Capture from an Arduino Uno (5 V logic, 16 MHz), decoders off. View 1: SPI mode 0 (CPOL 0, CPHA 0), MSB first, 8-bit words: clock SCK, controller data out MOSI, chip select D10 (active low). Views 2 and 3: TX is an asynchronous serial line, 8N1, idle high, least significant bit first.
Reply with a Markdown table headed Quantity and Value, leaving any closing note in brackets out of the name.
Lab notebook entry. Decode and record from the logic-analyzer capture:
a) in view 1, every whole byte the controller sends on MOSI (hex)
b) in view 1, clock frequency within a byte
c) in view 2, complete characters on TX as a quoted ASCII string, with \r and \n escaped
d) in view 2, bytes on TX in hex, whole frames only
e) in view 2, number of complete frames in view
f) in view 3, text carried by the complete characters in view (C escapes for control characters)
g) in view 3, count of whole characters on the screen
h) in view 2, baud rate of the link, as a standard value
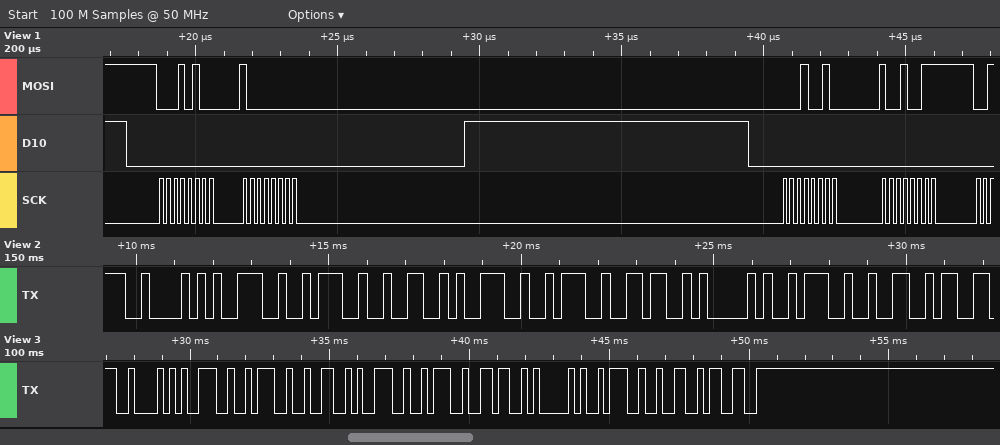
| Quantity | Value |
|---|---|
| in view 1, every whole byte the controller sends on MOSI | 14 80 12 93 |
| in view 1, clock frequency within a byte | 4 MHz |
| in view 2, complete characters on TX as a quoted ASCII string, with \r and \n escaped | "B9:29:6A:2" |
| in view 2, bytes on TX in hex, whole frames only | 42 39 3A 32 39 3A 36 41 3A 32 |
| in view 2, number of complete frames in view | 10 |
| in view 3, text carried by the complete characters in view | "B9:29:6A:23" |
| in view 3, count of whole characters on the screen | 11 |
| in view 2, baud rate of the link, as a standard value | 4800 baud |
